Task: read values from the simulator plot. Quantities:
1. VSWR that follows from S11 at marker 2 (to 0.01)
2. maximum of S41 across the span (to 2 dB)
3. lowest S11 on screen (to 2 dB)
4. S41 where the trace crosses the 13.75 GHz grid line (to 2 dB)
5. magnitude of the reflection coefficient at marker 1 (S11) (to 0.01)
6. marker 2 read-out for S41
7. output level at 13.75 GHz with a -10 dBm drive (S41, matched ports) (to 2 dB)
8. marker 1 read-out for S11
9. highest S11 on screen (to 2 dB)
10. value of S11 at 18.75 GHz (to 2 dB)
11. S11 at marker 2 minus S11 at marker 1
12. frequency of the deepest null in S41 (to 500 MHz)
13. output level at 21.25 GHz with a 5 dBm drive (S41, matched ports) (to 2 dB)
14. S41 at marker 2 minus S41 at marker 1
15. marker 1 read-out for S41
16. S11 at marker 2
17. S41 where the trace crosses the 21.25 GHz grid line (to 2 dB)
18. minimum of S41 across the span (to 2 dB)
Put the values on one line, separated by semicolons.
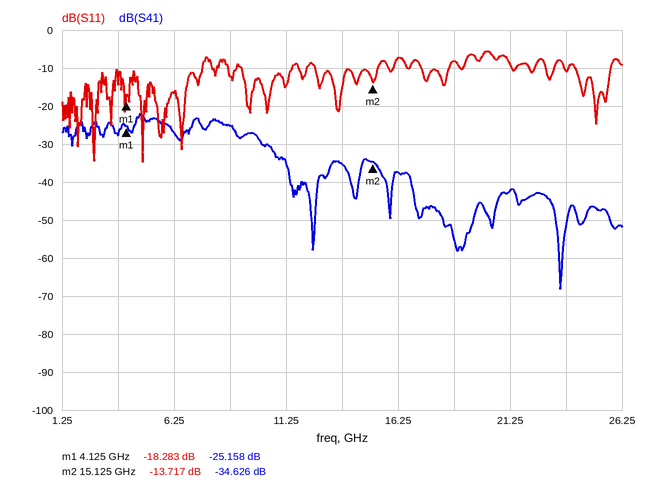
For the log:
1.52; -22 dB; -34 dB; -36 dB; 0.12; -34.626 dB; -46 dBm; -18.283 dB; -6 dB; -8 dB; 4.566 dB; 23.5 GHz; -38 dBm; -9.468 dB; -25.158 dB; -13.717 dB; -42 dB; -68 dB
